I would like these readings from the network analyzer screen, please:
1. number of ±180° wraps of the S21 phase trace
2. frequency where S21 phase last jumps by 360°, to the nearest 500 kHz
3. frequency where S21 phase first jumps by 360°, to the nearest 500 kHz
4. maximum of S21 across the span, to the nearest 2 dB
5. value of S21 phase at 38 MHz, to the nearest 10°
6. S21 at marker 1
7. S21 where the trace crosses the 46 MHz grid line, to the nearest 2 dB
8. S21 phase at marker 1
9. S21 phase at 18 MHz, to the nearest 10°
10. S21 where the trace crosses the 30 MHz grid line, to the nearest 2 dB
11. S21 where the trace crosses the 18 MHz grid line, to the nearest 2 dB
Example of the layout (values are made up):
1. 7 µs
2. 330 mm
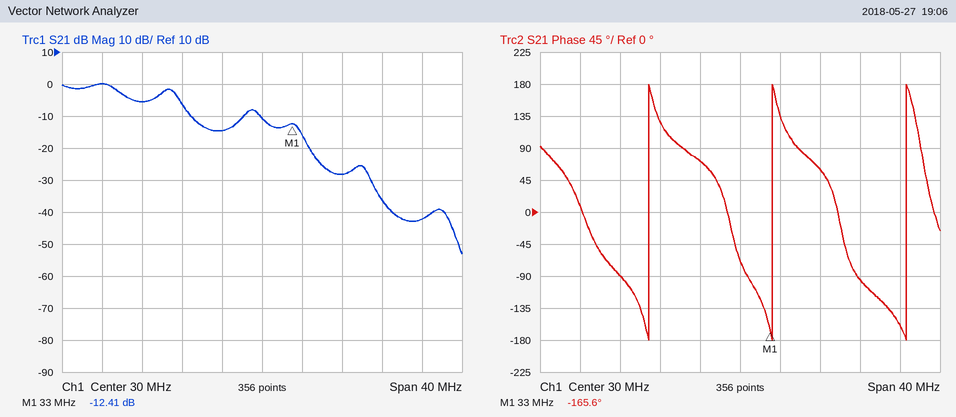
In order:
1. 3
2. 46.5 MHz
3. 21.0 MHz
4. 0 dB
5. 60°
6. -12.41 dB
7. -42 dB
8. -165.6°
9. -90°
10. -10 dB
11. -6 dB
